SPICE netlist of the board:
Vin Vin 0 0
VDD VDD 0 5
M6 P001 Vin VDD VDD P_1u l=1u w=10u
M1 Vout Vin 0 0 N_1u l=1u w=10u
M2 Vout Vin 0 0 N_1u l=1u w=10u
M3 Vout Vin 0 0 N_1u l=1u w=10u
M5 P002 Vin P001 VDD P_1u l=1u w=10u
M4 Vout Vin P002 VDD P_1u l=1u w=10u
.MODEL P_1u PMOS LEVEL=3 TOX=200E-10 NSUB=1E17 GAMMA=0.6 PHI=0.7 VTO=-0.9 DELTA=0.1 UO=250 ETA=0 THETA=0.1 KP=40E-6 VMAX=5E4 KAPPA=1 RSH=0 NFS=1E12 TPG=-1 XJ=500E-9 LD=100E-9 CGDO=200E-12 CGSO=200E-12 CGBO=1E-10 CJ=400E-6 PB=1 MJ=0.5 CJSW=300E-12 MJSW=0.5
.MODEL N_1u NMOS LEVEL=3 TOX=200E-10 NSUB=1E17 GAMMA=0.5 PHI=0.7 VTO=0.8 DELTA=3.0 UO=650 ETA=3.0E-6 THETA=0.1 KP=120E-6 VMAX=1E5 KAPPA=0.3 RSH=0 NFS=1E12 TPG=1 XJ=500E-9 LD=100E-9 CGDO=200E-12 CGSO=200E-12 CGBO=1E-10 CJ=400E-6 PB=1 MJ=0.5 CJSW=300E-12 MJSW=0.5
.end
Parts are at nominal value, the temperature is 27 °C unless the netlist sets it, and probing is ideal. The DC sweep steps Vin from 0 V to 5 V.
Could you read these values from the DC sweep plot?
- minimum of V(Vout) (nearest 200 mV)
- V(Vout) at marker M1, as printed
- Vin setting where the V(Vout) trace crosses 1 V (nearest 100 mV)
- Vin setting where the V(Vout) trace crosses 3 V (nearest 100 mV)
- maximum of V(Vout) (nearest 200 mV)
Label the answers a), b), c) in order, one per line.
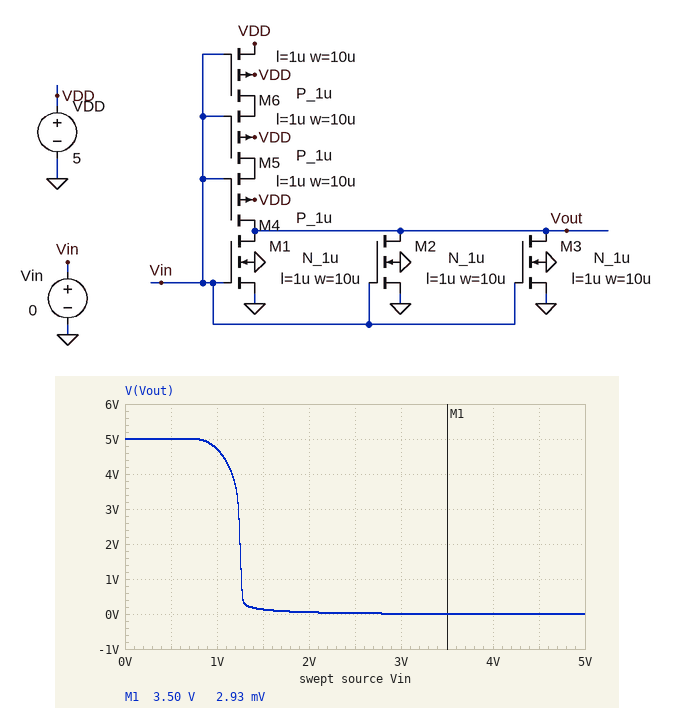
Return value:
a) 0 V
b) 2.93 mV
c) 1.3 V
d) 1.2 V
e) 5.0 V
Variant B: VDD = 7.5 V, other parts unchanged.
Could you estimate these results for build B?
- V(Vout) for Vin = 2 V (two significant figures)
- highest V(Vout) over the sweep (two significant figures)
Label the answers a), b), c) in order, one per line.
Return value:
a) 210 mV
b) 7.5 V
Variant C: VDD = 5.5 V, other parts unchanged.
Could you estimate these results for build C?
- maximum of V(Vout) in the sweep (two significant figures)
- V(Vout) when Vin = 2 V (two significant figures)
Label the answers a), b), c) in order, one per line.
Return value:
a) 5.5 V
b) 73 mV
